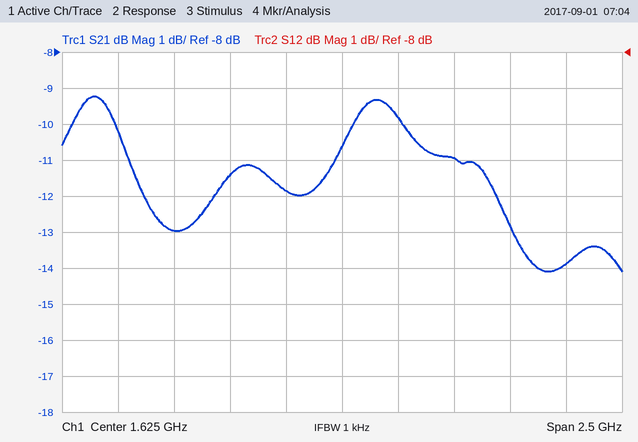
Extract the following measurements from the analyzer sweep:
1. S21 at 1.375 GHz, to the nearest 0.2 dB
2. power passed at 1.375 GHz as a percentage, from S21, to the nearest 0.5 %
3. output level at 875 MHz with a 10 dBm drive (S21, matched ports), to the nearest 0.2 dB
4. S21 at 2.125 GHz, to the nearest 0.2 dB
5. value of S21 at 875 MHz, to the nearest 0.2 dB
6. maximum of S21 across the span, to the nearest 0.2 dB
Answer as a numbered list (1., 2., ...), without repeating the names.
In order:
1. -11.8 dB
2. 6.5 %
3. -3.0 dBm
4. -11.0 dB
5. -13.0 dB
6. -9.2 dB
